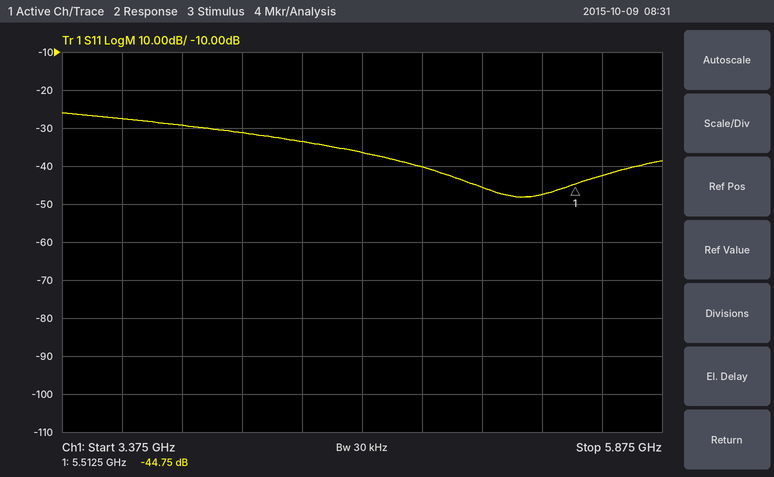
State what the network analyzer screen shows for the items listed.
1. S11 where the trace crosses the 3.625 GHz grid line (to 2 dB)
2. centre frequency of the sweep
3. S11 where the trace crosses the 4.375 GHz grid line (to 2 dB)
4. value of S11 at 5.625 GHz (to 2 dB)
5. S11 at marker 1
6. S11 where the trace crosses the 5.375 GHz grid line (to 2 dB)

-28 dB
4.625 GHz
-34 dB
-42 dB
-44.75 dB
-48 dB
